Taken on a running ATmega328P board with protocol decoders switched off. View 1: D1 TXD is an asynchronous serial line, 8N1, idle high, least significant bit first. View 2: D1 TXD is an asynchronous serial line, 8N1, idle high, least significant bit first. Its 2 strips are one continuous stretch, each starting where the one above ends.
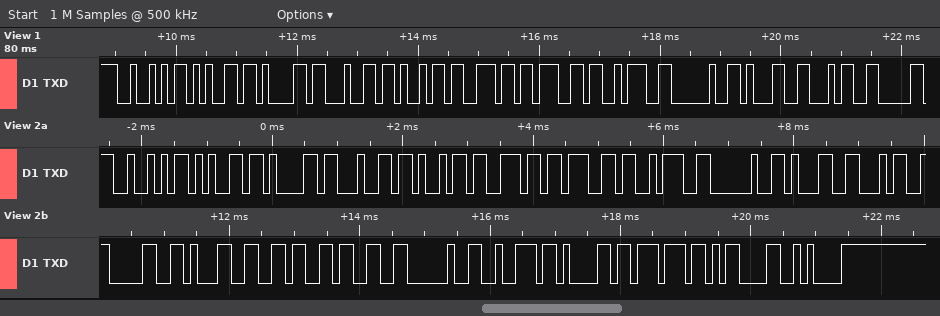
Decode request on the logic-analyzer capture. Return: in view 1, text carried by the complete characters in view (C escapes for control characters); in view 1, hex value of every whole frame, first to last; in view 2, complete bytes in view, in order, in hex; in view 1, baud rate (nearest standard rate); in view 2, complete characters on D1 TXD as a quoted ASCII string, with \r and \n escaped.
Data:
"Reading: 14"
52 65 61 64 69 6E 67 3A 20 31 34
52 65 61 64 69 6E 67 3A 20 31 34 30 31 36 33 20 72 61 77 0D 0A
9600 baud
"Reading: 140163 raw\r\n"
